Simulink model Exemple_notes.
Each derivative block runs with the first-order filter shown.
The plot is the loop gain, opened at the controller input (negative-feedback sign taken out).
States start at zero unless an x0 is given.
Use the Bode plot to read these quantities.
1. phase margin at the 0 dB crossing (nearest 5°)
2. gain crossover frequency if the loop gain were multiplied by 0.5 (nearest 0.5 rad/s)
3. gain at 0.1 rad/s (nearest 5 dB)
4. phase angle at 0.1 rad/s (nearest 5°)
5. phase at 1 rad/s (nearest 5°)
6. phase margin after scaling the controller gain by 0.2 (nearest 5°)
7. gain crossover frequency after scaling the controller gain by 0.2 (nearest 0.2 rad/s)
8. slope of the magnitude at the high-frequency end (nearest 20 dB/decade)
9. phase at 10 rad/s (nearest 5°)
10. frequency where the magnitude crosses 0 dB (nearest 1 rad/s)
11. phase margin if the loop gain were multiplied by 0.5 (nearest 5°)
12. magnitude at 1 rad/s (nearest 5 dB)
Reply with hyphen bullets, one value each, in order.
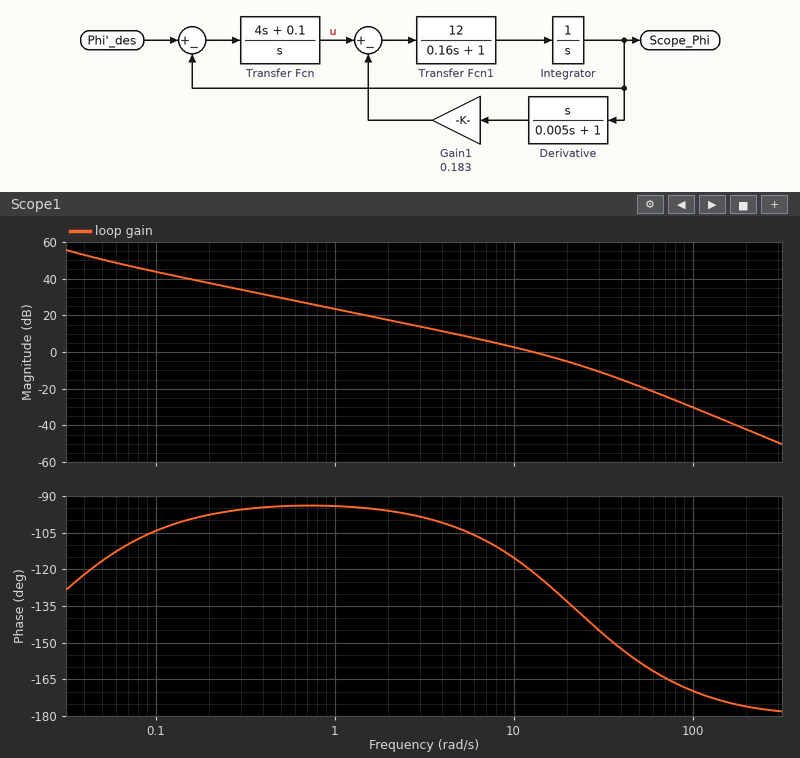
- 60°
- 7.0 rad/s
- 45 dB
- -105°
- -95°
- 80°
- 3.0 rad/s
- -40 dB/decade
- -115°
- 13 rad/s
- 70°
- 25 dB
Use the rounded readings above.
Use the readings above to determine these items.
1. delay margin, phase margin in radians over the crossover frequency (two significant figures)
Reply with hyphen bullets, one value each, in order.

- 0.081 s
